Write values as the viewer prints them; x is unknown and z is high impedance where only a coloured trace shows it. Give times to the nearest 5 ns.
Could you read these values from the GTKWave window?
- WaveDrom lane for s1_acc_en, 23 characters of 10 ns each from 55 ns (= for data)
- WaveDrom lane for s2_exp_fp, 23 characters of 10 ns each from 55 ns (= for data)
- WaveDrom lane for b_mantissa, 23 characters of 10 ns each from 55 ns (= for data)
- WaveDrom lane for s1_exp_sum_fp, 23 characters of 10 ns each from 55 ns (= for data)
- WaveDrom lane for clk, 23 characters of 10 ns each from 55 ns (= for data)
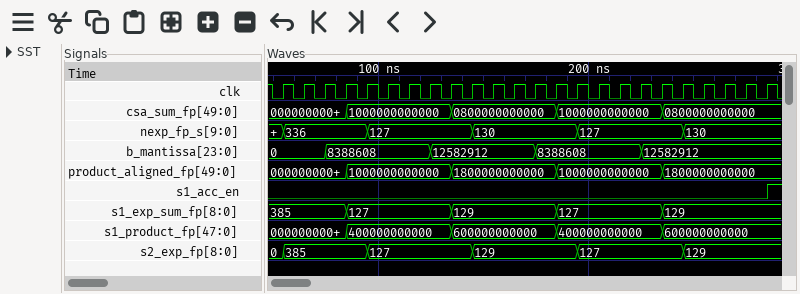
{name: 's1_acc_en', wave: '0......................'}
{name: 's2_exp_fp', wave: '=...=....=....=....=...', data: '385 127 129 127 129'}
{name: 'b_mantissa', wave: '=.=....=....=....=.....', data: '0 8388608 12582912 8388608 12582912'}
{name: 's1_exp_sum_fp', wave: '=..=....=....=....=....', data: '385 127 129 127 129'}
{name: 'clk', wave: 'p......................'}
